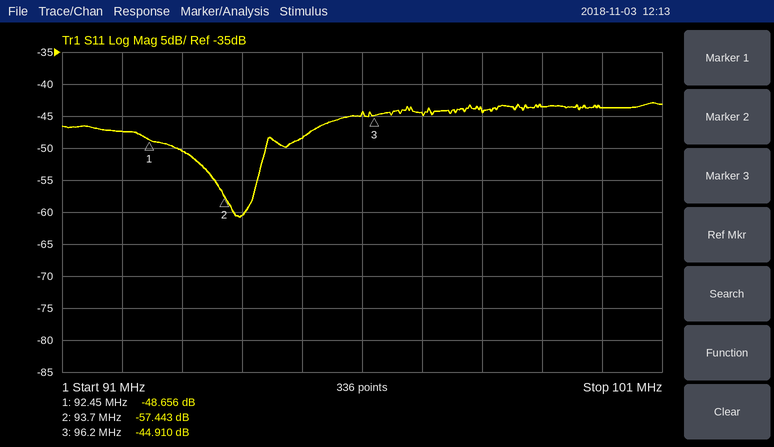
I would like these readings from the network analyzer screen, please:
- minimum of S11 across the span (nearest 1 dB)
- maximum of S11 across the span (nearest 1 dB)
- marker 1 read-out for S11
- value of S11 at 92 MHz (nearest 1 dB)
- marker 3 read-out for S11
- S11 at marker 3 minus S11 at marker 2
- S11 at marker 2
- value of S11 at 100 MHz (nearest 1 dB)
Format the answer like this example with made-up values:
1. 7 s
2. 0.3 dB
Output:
1. -61 dB
2. -43 dB
3. -48.656 dB
4. -47 dB
5. -44.910 dB
6. 12.533 dB
7. -57.443 dB
8. -44 dB
